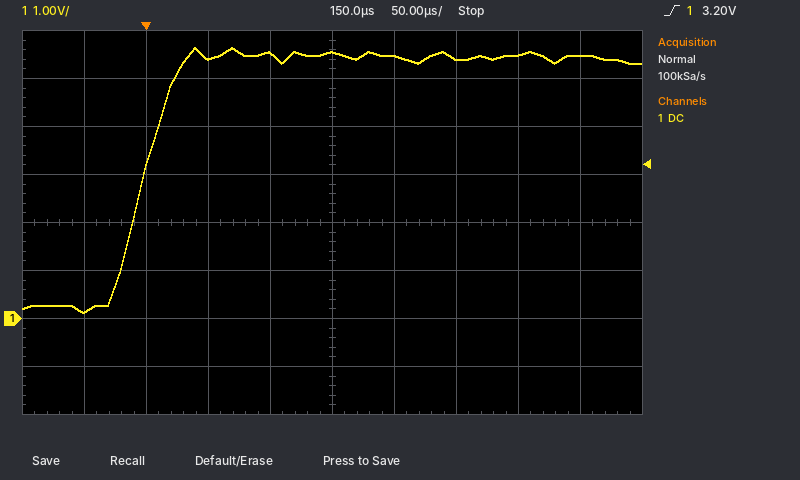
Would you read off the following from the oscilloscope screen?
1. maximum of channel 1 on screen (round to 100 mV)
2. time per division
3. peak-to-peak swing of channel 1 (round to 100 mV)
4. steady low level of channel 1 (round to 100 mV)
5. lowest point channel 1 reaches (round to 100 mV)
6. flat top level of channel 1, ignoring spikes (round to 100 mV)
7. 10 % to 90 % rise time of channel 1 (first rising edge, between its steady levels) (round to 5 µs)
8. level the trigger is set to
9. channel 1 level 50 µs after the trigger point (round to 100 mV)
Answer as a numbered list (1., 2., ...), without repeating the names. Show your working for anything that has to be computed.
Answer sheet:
1. 5.6 V
2. 50 µs
3. 5.6 V − (100 mV) = 5.5 V
4. 300 mV
5. 100 mV
6. 5.5 V
7. 45 µs
8. 3.20 V
9. 5.4 V
